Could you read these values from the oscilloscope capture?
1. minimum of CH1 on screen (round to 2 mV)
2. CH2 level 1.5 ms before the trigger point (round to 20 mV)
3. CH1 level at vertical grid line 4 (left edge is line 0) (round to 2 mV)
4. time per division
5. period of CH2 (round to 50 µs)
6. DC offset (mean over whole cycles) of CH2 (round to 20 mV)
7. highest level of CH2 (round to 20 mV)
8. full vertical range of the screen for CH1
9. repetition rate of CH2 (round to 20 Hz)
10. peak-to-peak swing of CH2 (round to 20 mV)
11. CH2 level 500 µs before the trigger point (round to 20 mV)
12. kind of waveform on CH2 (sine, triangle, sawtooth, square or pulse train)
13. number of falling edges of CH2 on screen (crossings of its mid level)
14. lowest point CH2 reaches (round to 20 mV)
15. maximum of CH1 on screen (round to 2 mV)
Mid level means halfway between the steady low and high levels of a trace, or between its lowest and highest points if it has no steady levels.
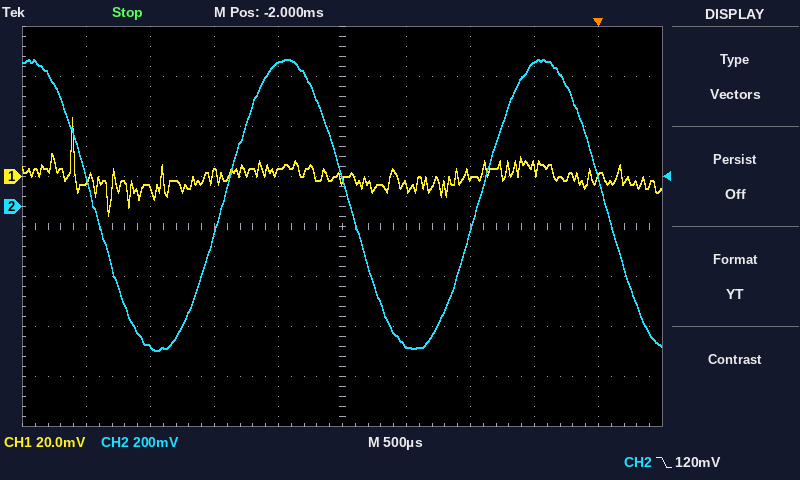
-16 mV
-560 mV
2 mV
500 µs
2.00 ms
0 mV
580 mV
160 mV
500 Hz
1.16 V
580 mV
sine
3
-580 mV
24 mV
